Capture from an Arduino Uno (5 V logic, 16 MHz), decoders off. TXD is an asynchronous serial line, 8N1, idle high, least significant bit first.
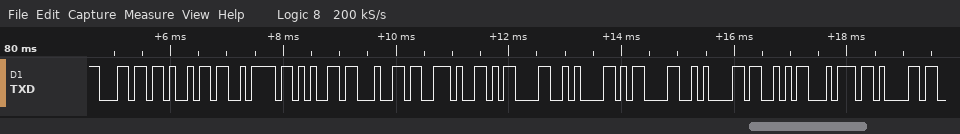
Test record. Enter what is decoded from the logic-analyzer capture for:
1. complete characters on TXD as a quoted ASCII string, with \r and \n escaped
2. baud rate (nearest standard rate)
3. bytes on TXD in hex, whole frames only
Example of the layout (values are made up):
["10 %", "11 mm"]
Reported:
["\"lized.\\r\\n\\r\\nSta\"", "9600 baud", "6C 69 7A 65 64 2E 0D 0A 0D 0A 53 74 61"]
